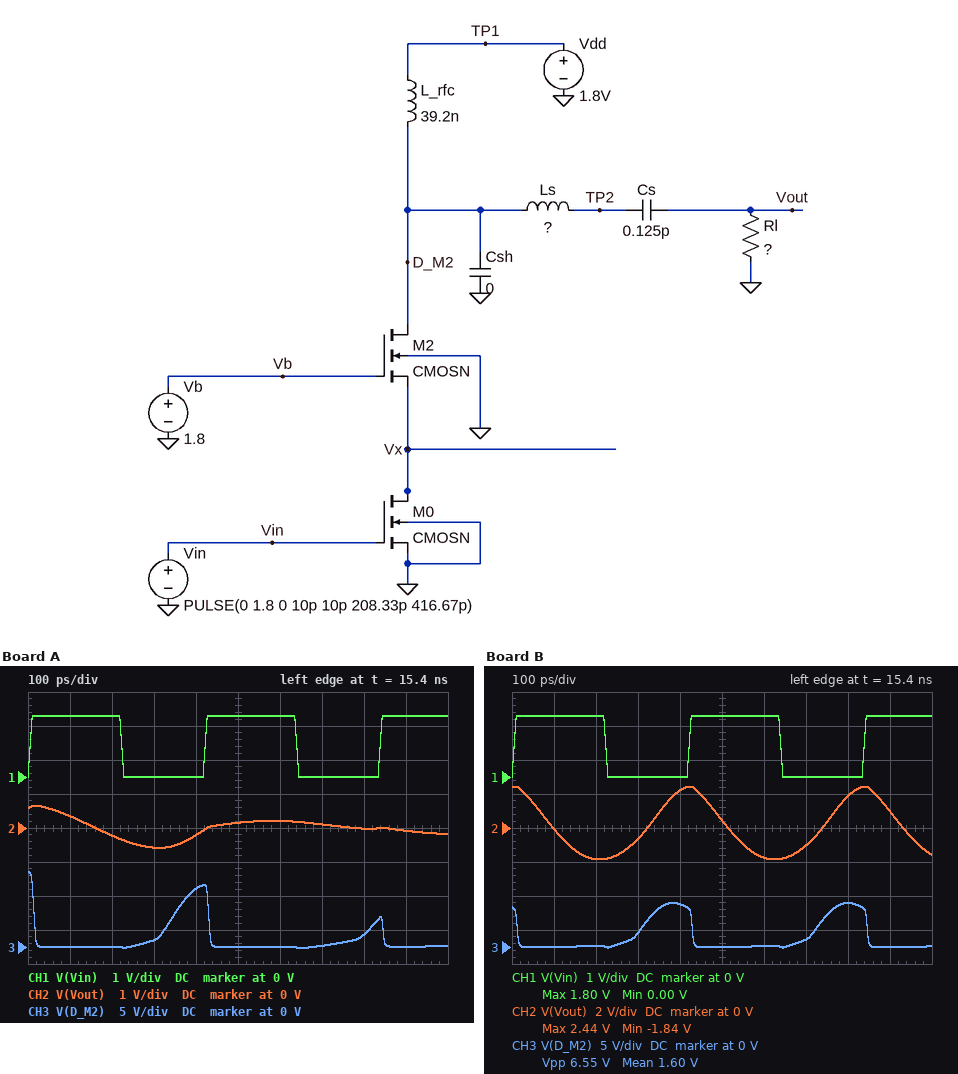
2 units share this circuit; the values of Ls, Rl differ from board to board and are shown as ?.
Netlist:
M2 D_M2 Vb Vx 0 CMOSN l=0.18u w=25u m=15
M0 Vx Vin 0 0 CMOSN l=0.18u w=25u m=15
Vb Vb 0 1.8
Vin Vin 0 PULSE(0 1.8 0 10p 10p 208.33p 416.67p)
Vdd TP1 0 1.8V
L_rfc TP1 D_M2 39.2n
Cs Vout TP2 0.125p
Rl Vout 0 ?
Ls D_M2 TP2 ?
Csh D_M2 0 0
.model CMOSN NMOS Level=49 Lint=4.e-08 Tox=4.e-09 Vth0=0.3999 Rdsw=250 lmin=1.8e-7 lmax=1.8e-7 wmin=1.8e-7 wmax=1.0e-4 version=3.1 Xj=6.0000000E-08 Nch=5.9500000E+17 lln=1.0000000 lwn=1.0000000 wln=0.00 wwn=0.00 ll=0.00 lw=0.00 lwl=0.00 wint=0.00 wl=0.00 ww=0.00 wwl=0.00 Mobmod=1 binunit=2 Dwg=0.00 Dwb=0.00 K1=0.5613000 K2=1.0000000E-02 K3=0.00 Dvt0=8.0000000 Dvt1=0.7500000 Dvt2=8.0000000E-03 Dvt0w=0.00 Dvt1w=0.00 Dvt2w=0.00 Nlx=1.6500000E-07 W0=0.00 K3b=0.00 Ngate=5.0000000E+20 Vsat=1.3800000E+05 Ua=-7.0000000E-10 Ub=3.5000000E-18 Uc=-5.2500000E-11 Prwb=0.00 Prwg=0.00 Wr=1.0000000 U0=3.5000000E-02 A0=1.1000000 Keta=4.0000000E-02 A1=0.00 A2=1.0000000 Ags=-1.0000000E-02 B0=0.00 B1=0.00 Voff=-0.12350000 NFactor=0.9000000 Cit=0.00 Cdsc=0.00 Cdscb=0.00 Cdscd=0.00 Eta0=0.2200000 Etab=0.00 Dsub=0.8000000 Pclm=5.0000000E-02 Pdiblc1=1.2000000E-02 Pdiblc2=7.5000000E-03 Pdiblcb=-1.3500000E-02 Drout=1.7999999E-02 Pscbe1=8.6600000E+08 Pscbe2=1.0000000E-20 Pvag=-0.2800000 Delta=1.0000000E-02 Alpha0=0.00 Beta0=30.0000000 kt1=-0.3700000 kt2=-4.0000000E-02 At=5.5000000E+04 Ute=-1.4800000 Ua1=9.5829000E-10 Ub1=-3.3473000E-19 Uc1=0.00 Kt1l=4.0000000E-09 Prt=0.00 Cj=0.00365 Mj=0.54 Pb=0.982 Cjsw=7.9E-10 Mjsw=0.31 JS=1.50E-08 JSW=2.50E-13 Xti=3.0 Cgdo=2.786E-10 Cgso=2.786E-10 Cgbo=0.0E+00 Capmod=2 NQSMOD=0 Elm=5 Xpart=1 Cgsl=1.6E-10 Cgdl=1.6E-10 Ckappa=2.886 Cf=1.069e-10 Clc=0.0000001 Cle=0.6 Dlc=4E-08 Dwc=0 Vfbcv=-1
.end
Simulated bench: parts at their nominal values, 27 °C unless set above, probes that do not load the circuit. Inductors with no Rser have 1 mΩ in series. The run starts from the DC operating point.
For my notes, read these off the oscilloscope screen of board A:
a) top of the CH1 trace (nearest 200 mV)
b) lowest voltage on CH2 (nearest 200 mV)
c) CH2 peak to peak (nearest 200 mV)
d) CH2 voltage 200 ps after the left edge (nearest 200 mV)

1.8 V
-600 mV
1.2 V
-200 mV
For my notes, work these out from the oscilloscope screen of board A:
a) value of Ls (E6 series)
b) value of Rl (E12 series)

100 nH
68 Ω
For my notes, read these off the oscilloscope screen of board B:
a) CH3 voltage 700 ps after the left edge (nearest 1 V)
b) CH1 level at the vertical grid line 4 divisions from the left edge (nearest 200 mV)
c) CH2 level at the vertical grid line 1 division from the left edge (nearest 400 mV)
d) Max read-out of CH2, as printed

1 V
0 V
0 V
2.44 V
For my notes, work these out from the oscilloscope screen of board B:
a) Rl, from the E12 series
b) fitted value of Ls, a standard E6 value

180 Ω
47 nH
